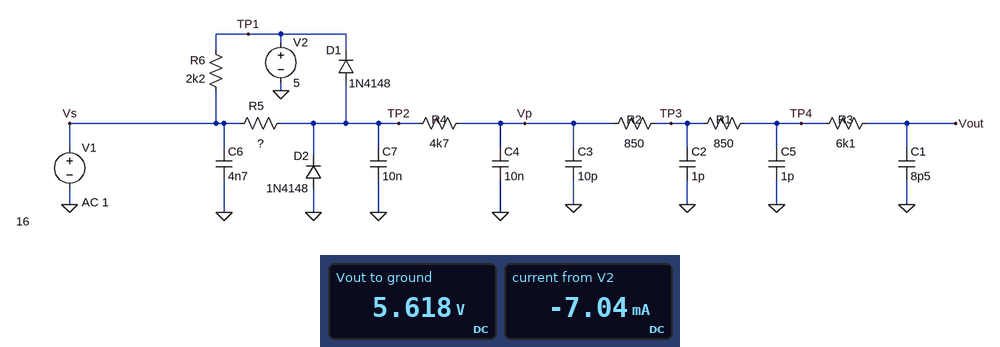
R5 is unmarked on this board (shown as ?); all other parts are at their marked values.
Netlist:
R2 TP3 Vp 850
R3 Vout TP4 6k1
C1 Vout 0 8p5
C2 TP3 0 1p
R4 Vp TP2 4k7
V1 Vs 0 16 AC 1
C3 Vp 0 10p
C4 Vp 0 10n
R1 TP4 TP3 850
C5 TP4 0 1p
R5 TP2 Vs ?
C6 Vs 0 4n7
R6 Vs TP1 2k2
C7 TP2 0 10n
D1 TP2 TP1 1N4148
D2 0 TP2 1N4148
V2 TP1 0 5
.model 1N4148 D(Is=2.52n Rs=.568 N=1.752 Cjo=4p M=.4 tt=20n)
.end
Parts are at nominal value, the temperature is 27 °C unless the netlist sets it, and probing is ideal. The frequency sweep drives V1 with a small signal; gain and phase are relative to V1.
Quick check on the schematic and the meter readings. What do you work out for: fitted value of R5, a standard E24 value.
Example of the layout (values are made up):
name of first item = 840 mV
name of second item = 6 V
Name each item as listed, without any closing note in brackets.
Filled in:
fitted value of R5, a standard E24 value = 5.1 kΩ
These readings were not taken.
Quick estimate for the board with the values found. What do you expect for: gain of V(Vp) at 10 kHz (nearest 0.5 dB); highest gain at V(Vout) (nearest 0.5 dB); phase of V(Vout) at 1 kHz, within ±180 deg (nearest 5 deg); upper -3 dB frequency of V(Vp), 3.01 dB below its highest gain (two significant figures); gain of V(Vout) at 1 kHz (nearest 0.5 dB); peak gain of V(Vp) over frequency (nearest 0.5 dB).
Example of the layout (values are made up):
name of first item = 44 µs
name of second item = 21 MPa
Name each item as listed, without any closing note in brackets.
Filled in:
gain of V(Vp) at 10 kHz = -57.0 dB
highest gain at V(Vout) = -47.0 dB
phase of V(Vout) at 1 kHz, within ±180 deg = -15 deg
upper -3 dB frequency of V(Vp), 3.01 dB below its highest gain = 3.4 kHz
gain of V(Vout) at 1 kHz = -47.5 dB
peak gain of V(Vp) over frequency = -47.0 dB
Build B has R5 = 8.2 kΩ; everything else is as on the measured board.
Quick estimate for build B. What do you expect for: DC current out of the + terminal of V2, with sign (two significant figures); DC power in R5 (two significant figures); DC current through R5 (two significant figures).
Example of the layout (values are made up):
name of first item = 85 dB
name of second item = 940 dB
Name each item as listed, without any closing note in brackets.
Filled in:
DC current out of the + terminal of V2, with sign = -6.3 mA
DC power in R5 = 13 mW
DC current through R5 = 1.3 mA
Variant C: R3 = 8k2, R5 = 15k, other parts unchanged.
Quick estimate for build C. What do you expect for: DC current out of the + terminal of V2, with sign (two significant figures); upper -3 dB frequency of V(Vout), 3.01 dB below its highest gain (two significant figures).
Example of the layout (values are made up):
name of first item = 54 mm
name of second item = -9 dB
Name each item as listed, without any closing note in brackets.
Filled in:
DC current out of the + terminal of V2, with sign = -5.7 mA
upper -3 dB frequency of V(Vout), 3.01 dB below its highest gain = 3.3 kHz
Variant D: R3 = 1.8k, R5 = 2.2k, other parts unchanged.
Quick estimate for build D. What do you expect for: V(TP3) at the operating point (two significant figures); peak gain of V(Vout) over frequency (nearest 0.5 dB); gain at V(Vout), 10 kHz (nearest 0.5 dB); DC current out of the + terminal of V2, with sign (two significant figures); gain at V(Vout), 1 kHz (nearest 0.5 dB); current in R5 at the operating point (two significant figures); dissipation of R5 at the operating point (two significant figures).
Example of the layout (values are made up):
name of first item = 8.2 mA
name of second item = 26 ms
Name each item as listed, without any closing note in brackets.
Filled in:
V(TP3) at the operating point = 5.7 V
peak gain of V(Vout) over frequency = -46.5 dB
gain at V(Vout), 10 kHz = -56.5 dB
DC current out of the + terminal of V2, with sign = -9.7 mA
gain at V(Vout), 1 kHz = -47.0 dB
current in R5 at the operating point = 4.7 mA
dissipation of R5 at the operating point = 49 mW
